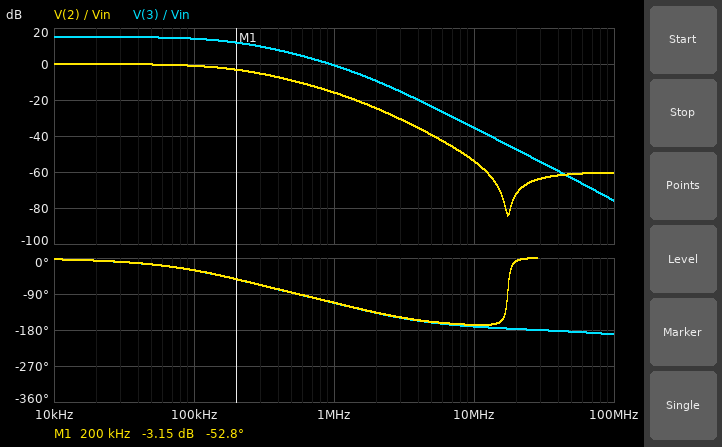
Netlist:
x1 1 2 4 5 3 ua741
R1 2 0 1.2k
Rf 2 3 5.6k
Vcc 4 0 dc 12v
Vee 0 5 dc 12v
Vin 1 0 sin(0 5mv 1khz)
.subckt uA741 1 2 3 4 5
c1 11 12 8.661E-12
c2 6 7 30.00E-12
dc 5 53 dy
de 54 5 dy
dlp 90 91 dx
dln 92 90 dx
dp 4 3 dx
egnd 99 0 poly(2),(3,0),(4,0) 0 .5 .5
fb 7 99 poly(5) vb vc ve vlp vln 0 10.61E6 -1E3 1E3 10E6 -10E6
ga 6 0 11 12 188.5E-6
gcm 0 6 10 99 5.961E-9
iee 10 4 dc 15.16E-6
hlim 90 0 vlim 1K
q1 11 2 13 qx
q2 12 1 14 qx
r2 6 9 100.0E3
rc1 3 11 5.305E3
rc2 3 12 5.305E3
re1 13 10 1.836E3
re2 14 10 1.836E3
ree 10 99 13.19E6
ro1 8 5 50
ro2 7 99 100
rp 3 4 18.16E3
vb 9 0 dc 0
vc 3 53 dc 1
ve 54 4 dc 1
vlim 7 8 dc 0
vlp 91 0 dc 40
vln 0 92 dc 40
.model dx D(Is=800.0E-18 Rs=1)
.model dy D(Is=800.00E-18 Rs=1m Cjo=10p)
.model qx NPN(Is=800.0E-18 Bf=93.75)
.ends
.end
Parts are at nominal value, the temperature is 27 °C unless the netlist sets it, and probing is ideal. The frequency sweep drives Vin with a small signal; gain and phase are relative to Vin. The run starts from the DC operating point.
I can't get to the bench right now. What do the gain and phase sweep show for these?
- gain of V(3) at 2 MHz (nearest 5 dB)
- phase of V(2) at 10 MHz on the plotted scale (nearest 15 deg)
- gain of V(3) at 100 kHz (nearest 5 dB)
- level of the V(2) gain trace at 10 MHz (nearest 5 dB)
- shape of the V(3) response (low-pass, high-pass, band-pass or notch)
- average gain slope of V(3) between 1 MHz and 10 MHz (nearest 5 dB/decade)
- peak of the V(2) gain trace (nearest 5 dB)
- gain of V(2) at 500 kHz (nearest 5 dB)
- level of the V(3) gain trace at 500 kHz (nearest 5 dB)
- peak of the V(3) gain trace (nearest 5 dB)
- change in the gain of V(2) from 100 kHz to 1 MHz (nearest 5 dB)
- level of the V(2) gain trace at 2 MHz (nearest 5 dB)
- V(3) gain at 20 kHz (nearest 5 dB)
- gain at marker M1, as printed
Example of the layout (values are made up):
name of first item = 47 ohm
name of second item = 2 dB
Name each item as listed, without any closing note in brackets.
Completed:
gain of V(3) at 2 MHz = -10 dB
phase of V(2) at 10 MHz on the plotted scale = -165 deg
gain of V(3) at 100 kHz = 15 dB
level of the V(2) gain trace at 10 MHz = -55 dB
shape of the V(3) response = low-pass
average gain slope of V(3) between 1 MHz and 10 MHz = -35 dB/decade
peak of the V(2) gain trace = 0 dB
gain of V(2) at 500 kHz = -10 dB
level of the V(3) gain trace at 500 kHz = 5 dB
peak of the V(3) gain trace = 15 dB
change in the gain of V(2) from 100 kHz to 1 MHz = -15 dB
level of the V(2) gain trace at 2 MHz = -25 dB
V(3) gain at 20 kHz = 15 dB
gain at marker M1, as printed = -3.15 dB
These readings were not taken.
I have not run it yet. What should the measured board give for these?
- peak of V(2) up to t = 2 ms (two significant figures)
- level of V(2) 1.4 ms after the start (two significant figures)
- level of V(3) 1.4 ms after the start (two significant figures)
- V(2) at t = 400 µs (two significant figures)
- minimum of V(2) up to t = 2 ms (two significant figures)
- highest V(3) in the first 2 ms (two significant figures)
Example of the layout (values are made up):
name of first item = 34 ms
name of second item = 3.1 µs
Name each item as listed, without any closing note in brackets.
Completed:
peak of V(2) up to t = 2 ms = 5.0 mV
level of V(2) 1.4 ms after the start = 3.0 mV
level of V(3) 1.4 ms after the start = 17 mV
V(2) at t = 400 µs = 3.0 mV
minimum of V(2) up to t = 2 ms = -5.0 mV
highest V(3) in the first 2 ms = 29 mV
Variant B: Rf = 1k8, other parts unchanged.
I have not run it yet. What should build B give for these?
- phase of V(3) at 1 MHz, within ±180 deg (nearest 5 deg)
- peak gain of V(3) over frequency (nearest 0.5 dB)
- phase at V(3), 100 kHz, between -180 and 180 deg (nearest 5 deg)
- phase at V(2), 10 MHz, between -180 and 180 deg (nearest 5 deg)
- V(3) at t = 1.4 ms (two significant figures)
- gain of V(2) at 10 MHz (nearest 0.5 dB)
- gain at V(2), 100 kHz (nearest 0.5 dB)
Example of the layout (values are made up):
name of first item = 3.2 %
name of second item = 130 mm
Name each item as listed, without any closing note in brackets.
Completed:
phase of V(3) at 1 MHz, within ±180 deg = -100 deg
peak gain of V(3) over frequency = 8.0 dB
phase at V(3), 100 kHz, between -180 and 180 deg = -15 deg
phase at V(2), 10 MHz, between -180 and 180 deg = -170 deg
V(3) at t = 1.4 ms = 7.6 mV
gain of V(2) at 10 MHz = -44.5 dB
gain at V(2), 100 kHz = 0 dB
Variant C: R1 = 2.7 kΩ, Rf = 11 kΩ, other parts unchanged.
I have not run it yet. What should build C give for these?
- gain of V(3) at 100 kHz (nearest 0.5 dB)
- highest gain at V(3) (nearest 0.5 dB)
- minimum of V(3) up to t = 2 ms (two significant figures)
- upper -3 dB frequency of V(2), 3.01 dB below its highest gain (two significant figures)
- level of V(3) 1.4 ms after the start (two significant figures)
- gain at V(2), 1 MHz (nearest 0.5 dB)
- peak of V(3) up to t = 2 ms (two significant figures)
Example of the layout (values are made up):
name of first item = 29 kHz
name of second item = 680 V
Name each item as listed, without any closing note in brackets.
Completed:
gain of V(3) at 100 kHz = 13.5 dB
highest gain at V(3) = 14.0 dB
minimum of V(3) up to t = 2 ms = -24 mV
upper -3 dB frequency of V(2), 3.01 dB below its highest gain = 220 kHz
level of V(3) 1.4 ms after the start = 16 mV
gain at V(2), 1 MHz = -15.0 dB
peak of V(3) up to t = 2 ms = 26 mV
